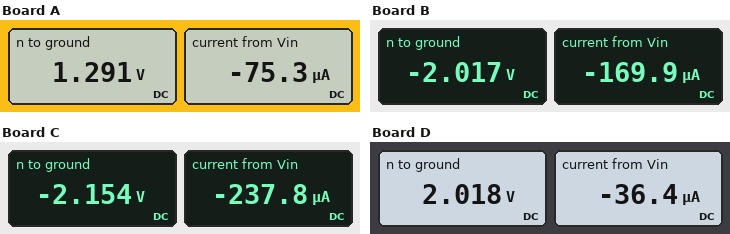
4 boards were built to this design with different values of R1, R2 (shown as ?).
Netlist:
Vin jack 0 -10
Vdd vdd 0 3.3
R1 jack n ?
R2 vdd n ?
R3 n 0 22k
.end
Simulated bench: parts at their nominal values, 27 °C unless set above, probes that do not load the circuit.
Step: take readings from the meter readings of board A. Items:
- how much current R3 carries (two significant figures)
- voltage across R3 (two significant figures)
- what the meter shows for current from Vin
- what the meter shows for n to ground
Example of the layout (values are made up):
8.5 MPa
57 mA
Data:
59 µA
1.3 V
-75.3 µA
1.291 V
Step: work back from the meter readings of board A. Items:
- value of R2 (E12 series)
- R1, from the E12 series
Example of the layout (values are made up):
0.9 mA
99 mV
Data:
15 kΩ
150 kΩ
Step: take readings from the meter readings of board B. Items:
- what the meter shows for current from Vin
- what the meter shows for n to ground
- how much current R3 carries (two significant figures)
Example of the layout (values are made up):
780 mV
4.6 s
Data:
-169.9 µA
-2.017 V
92 µA
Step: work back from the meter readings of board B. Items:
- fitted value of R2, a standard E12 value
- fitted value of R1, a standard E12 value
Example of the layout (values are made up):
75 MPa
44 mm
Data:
68 kΩ
47 kΩ
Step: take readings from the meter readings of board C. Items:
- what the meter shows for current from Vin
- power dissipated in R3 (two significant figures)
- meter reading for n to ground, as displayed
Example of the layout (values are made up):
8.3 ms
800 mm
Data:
-237.8 µA
210 µW
-2.154 V
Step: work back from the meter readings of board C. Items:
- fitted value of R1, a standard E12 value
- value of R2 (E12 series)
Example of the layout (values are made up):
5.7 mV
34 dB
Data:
33 kΩ
39 kΩ
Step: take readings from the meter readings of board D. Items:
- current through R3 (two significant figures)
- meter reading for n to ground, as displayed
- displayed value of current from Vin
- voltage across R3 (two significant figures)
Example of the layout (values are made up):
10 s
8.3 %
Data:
92 µA
2.018 V
-36.4 µA
2.0 V
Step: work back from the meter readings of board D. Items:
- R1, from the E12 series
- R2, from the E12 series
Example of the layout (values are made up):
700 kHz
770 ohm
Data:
330 kΩ
10 kΩ
